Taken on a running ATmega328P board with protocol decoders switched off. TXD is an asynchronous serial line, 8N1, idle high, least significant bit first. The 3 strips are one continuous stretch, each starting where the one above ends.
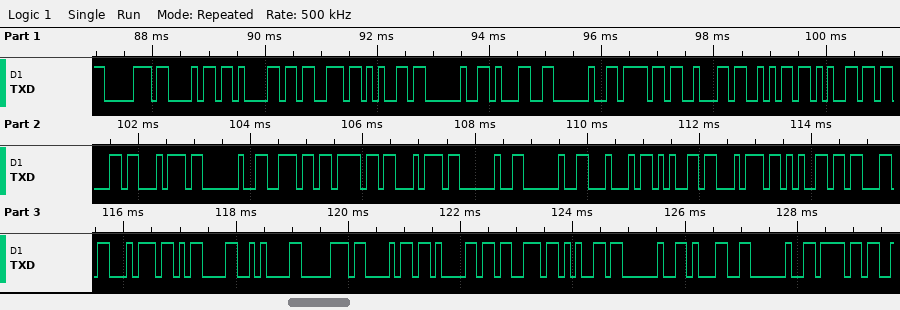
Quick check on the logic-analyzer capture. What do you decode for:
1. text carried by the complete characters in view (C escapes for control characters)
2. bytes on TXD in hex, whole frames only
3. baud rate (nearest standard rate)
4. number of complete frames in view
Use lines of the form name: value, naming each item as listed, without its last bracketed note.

text carried by the complete characters in view: "phase 1 object not  Detect\r\nphase 1 o"
bytes on TXD in hex, whole frames only: 70 68 61 73 65 20 31 20 6F 62 6A 65 63 74 20 6E 6F 74 20 20 44 65 74 65 63 74 0D 0A 70 68 61 73 65 20 31 20 6F
baud rate: 9600 baud
number of complete frames in view: 37
